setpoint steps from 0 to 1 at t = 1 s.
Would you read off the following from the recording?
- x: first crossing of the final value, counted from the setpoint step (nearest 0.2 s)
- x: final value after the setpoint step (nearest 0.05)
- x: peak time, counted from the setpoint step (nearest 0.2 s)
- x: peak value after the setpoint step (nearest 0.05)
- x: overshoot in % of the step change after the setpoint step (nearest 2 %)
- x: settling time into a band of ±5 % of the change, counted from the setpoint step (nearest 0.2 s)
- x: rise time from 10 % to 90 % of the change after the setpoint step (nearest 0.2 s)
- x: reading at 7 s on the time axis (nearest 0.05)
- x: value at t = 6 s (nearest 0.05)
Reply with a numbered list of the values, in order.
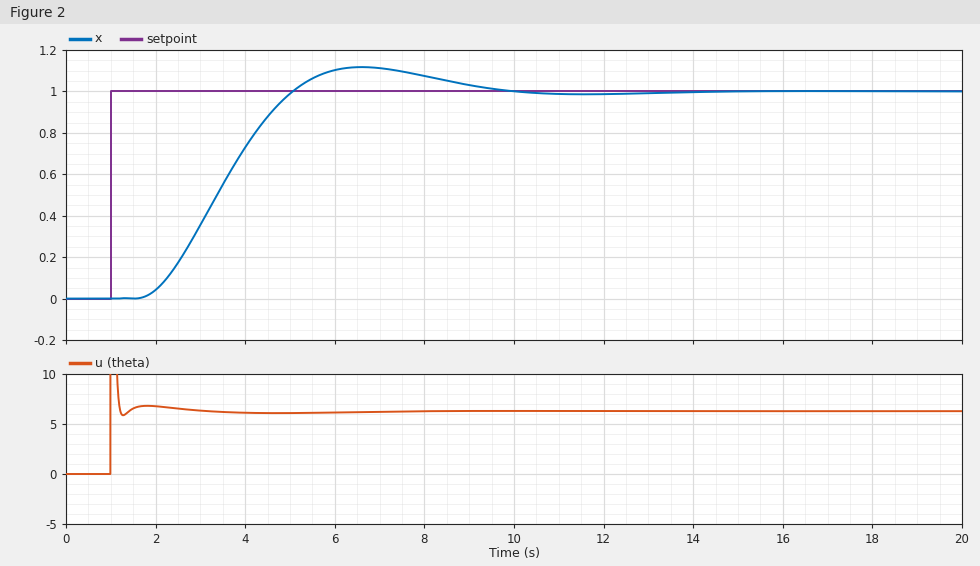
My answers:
1. 4.0 s
2. 1.00
3. 5.6 s
4. 1.10
5. 12 %
6. 7.6 s
7. 2.4 s
8. 1.10
9. 1.10
